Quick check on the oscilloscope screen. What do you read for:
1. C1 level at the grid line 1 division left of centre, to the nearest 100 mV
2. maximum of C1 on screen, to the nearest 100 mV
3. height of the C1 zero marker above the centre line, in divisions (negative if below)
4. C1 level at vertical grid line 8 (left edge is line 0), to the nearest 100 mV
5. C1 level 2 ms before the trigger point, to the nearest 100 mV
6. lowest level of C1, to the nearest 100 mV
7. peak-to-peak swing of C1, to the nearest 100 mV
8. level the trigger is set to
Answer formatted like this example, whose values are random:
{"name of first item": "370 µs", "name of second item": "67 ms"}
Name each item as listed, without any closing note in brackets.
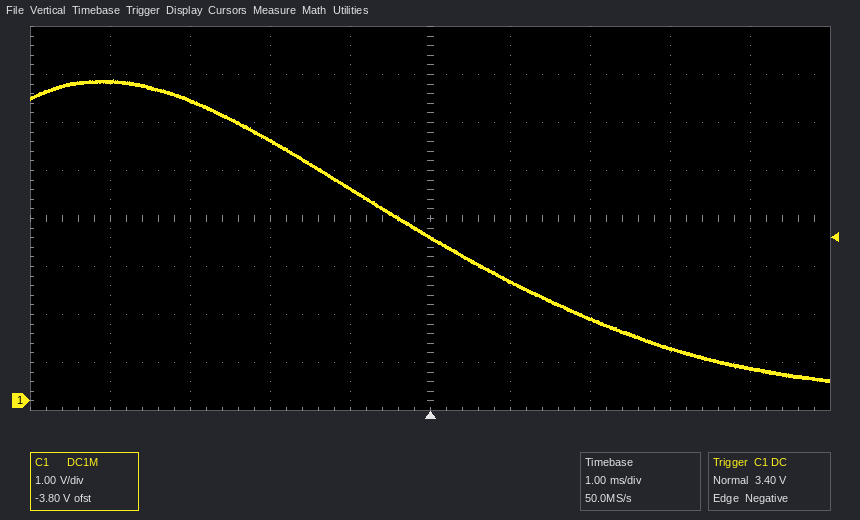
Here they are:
{"C1 level at the grid line 1 division left of centre, to the nearest 100 mV": "4.4 V", "maximum of C1 on screen, to the nearest 100 mV": "6.7 V", "height of the C1 zero marker above the centre line, in divisions": "-3.8 div", "C1 level at vertical grid line 8 (left edge is line 0), to the nearest 100 mV": "1.1 V", "C1 level 2 ms before the trigger point, to the nearest 100 mV": "5.4 V", "lowest level of C1, to the nearest 100 mV": "400 mV", "peak-to-peak swing of C1, to the nearest 100 mV": "6.3 V", "level the trigger is set to": "3.40 V"}
